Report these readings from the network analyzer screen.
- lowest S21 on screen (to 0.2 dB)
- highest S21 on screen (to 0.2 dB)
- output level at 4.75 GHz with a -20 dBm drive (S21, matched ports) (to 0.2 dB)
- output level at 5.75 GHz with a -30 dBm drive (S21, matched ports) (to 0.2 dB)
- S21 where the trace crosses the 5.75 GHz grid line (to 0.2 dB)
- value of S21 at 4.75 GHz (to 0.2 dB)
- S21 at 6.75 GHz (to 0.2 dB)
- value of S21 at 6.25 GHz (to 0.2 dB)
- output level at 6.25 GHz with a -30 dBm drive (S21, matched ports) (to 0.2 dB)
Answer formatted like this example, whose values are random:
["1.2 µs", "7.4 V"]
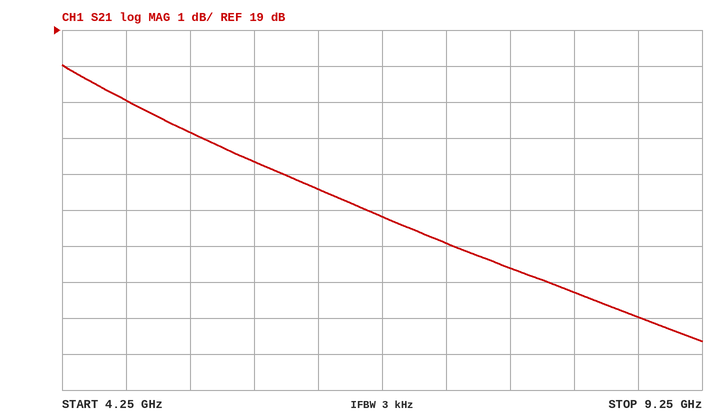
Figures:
["10.4 dB", "18.0 dB", "-3.0 dBm", "-14.6 dBm", "15.4 dB", "17.0 dB", "13.8 dB", "14.6 dB", "-15.4 dBm"]
